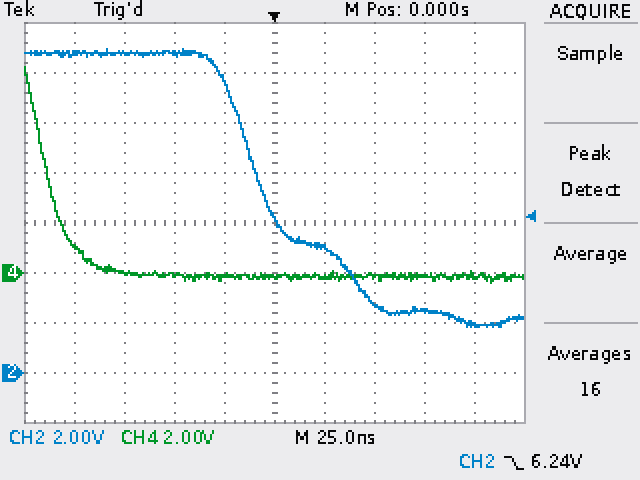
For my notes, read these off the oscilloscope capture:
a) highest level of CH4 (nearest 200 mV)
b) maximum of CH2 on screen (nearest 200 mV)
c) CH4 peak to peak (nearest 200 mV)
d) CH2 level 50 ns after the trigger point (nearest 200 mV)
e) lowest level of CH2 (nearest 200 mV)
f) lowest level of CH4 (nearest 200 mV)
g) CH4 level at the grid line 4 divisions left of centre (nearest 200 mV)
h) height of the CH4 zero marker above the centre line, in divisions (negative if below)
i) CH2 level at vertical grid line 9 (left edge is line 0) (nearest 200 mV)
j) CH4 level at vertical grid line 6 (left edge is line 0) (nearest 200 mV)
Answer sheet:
8.2 V
13.0 V
8.6 V
2.8 V
1.8 V
-400 mV
1.2 V
-1.0 div
2.0 V
-200 mV
